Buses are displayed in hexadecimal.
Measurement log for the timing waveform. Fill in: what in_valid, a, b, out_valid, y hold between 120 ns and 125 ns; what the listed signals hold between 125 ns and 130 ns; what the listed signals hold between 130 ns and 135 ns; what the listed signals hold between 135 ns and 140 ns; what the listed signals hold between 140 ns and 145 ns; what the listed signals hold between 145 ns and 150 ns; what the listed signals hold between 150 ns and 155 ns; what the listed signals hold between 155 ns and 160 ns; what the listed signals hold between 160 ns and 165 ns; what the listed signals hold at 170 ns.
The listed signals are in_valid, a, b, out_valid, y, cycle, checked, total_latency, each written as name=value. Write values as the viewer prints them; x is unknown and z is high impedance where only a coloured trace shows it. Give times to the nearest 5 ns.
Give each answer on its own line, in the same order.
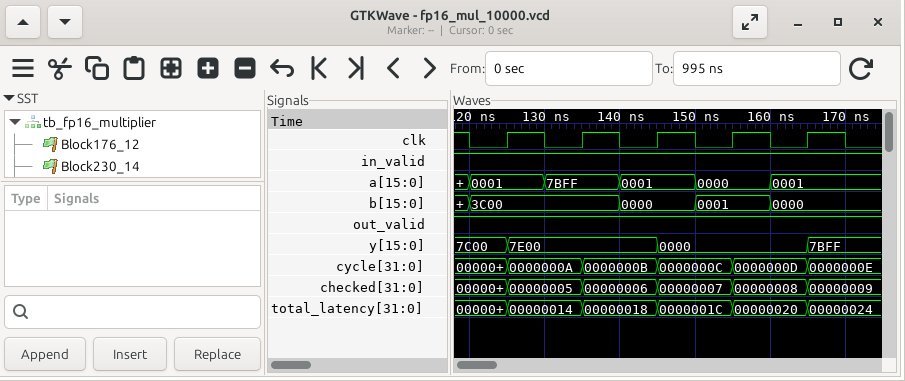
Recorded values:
in_valid=1, a=0001, b=3C00, out_valid=1, y=7C00
in_valid=1, a=0001, b=3C00, out_valid=1, y=7E00, cycle=0000000A, checked=00000005, total_latency=00000014
in_valid=1, a=7BFF, b=3C00, out_valid=1, y=7E00, cycle=0000000A, checked=00000005, total_latency=00000014
in_valid=1, a=7BFF, b=3C00, out_valid=1, y=7E00, cycle=0000000B, checked=00000006, total_latency=00000018
in_valid=1, a=0001, b=0000, out_valid=1, y=7E00, cycle=0000000B, checked=00000006, total_latency=00000018
in_valid=1, a=0001, b=0000, out_valid=1, y=0000, cycle=0000000C, checked=00000007, total_latency=0000001C
in_valid=1, a=0000, b=0001, out_valid=1, y=0000, cycle=0000000C, checked=00000007, total_latency=0000001C
in_valid=1, a=0000, b=0001, out_valid=1, y=0000, cycle=0000000D, checked=00000008, total_latency=00000020
in_valid=1, a=0001, b=0000, out_valid=1, y=0000, cycle=0000000D, checked=00000008, total_latency=00000020
in_valid=1, a=0001, b=0000, out_valid=1, y=7BFF, cycle=0000000E, checked=00000009, total_latency=00000024
